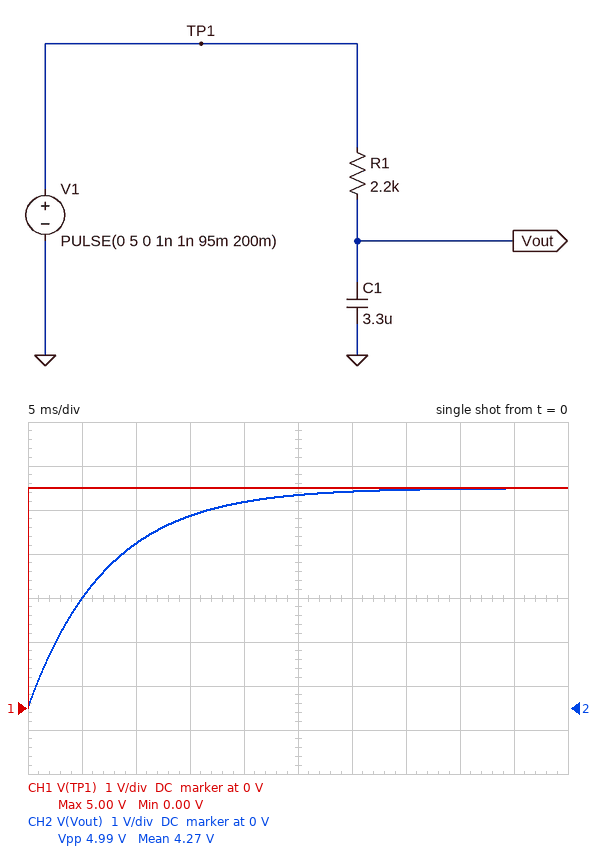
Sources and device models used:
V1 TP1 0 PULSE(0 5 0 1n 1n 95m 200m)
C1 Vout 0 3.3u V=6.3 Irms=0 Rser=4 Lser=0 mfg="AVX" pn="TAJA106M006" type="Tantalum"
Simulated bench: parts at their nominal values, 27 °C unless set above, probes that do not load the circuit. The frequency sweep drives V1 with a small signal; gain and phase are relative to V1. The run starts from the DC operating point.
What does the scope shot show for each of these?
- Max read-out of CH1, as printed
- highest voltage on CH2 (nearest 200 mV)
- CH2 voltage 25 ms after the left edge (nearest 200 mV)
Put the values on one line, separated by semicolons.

5.00 V; 5.0 V; 4.8 V
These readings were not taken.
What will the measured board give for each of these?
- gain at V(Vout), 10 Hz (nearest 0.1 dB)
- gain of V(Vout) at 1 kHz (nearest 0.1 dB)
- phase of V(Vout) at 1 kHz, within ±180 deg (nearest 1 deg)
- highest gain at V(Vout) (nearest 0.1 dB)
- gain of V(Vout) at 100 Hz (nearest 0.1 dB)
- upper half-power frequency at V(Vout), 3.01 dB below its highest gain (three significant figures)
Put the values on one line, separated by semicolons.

-0.8 dB; -33.2 dB; -84 deg; 0 dB; -13.4 dB; 21.9 Hz
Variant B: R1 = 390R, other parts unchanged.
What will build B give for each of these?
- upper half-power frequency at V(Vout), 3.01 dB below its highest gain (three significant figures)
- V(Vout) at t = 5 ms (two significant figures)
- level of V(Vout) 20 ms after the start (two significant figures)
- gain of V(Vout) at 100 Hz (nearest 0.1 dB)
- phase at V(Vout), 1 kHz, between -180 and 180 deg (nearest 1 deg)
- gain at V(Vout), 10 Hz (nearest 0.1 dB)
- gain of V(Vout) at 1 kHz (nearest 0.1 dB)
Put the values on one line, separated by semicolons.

122 Hz; 4.9 V; 5.0 V; -2.2 dB; -78 deg; 0 dB; -18.3 dB
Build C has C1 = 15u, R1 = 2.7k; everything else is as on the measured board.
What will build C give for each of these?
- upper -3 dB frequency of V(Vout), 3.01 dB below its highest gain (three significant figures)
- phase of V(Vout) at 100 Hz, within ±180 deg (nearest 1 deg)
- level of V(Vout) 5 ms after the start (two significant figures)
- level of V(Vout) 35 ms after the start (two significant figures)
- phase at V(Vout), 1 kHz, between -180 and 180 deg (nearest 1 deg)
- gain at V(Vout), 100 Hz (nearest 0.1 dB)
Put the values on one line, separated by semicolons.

3.92 Hz; -86 deg; 590 mV; 2.9 V; -69 deg; -28.1 dB
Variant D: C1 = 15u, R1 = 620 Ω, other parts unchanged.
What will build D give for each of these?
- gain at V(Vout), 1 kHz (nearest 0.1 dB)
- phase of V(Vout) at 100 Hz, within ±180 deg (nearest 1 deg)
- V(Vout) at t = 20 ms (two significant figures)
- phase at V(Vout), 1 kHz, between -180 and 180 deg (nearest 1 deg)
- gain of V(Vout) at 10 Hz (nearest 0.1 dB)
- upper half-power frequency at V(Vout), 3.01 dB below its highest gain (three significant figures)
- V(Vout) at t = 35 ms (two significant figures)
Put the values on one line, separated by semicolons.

-34.8 dB; -78 deg; 4.4 V; -68 deg; -1.3 dB; 17.0 Hz; 4.9 V
